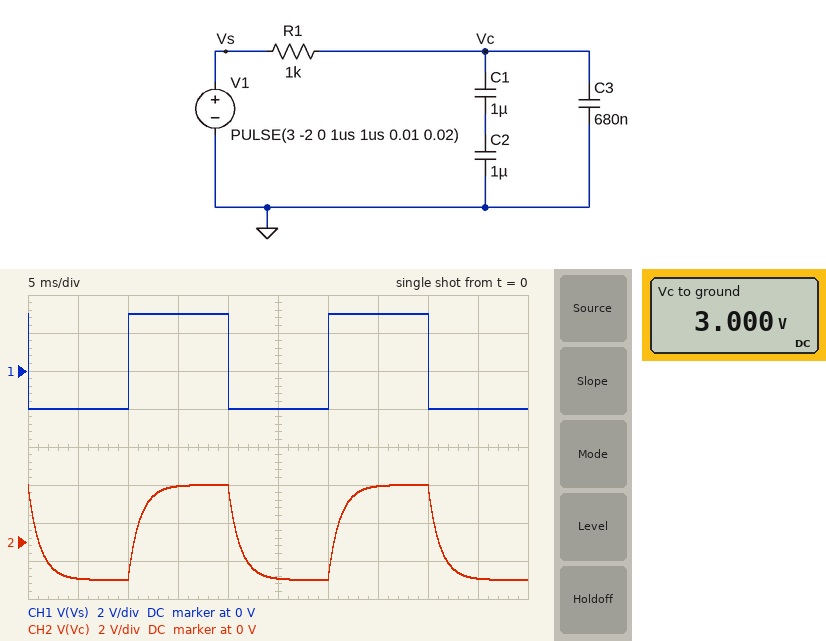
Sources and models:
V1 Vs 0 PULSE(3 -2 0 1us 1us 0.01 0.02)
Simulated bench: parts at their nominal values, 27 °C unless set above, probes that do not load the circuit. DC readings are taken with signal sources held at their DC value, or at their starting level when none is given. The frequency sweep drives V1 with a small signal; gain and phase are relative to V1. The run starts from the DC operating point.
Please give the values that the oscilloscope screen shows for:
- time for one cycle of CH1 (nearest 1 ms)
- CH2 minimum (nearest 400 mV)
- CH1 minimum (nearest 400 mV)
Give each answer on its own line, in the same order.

20 ms
-2.0 V
-2.0 V
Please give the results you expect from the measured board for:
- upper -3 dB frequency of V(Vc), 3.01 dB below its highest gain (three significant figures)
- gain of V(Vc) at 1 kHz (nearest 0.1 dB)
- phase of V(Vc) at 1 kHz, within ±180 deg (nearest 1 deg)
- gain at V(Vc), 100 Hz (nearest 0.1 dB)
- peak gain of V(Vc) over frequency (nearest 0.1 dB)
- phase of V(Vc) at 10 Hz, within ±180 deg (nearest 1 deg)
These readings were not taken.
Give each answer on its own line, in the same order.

135 Hz
-17.5 dB
-82 deg
-1.9 dB
0 dB
-4 deg
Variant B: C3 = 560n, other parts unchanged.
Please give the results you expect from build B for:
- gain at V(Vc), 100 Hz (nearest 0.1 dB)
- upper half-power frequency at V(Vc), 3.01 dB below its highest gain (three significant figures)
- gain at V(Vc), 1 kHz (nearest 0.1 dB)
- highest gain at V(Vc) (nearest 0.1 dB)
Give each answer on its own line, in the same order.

-1.6 dB
150 Hz
-16.6 dB
0 dB
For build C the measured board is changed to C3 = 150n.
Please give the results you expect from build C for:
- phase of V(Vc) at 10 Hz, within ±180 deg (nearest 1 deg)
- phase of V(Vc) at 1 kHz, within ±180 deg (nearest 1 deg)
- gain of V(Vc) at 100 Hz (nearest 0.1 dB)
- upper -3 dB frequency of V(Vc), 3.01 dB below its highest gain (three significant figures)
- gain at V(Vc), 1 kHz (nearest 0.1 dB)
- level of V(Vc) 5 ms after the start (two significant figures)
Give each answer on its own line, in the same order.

-2 deg
-76 deg
-0.7 dB
245 Hz
-12.5 dB
-2.0 V
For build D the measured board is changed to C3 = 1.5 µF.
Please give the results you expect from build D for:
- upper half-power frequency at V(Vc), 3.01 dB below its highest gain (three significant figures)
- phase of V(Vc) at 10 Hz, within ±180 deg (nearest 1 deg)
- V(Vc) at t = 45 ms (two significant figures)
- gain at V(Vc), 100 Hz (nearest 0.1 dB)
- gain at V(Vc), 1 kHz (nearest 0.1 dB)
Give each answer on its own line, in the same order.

79.6 Hz
-7 deg
-1.6 V
-4.1 dB
-22.0 dB
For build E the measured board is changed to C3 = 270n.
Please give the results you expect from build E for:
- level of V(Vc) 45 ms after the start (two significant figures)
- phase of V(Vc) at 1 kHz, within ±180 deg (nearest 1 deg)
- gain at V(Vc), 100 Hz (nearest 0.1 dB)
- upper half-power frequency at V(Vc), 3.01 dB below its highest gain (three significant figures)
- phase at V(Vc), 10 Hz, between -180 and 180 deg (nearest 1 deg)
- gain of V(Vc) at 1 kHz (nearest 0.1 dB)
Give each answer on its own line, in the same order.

-2.0 V
-78 deg
-0.9 dB
207 Hz
-3 deg
-13.9 dB
